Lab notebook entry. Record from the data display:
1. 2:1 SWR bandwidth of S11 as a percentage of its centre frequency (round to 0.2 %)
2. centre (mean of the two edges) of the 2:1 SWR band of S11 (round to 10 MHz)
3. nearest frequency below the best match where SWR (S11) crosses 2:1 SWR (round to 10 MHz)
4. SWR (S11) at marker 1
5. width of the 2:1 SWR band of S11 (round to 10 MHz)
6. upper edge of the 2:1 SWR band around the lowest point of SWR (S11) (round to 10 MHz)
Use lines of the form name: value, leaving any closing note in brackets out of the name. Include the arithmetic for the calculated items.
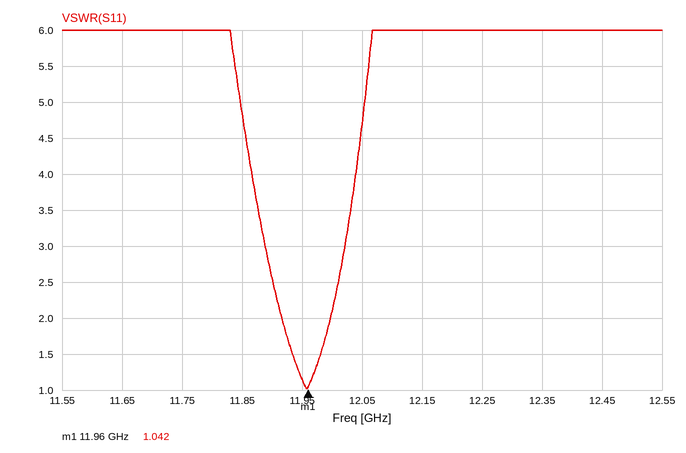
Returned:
2:1 SWR bandwidth of S11 as a percentage of its centre frequency: 80 MHz / 11.96 GHz ≈ 0.669 %, so 0.6 % to the nearest 0.2 %
centre (mean of the two edges) of the 2:1 SWR band of S11: 11.96 GHz
nearest frequency below the best match where SWR (S11) crosses 2:1 SWR: 11.92 GHz
SWR (S11) at marker 1: 1.042
width of the 2:1 SWR band of S11: 12.00 GHz − 11.92 GHz = 80 MHz
upper edge of the 2:1 SWR band around the lowest point of SWR (S11): 12.00 GHz
